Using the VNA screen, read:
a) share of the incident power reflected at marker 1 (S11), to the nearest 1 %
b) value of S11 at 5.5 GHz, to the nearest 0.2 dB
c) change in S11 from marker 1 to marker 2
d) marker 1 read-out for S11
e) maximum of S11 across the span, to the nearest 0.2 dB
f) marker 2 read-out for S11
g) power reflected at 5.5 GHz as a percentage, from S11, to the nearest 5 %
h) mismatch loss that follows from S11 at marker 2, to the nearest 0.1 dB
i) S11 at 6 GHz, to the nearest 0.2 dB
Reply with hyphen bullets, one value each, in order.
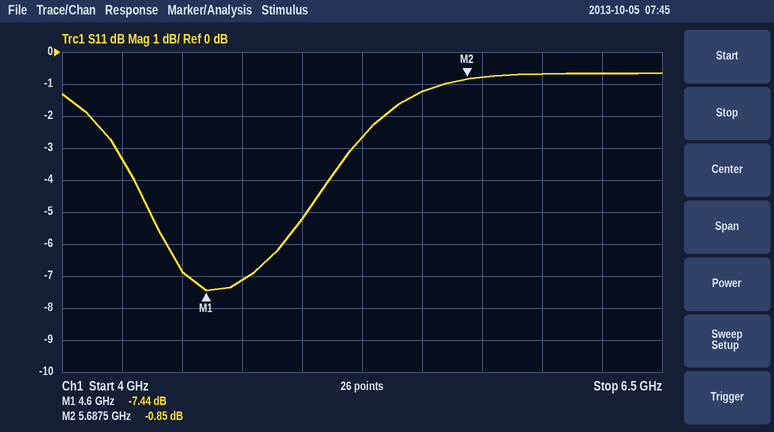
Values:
- 18 %
- -1.2 dB
- 6.59 dB
- -7.44 dB
- -0.6 dB
- -0.85 dB
- 75 %
- 7.5 dB
- -0.6 dB
